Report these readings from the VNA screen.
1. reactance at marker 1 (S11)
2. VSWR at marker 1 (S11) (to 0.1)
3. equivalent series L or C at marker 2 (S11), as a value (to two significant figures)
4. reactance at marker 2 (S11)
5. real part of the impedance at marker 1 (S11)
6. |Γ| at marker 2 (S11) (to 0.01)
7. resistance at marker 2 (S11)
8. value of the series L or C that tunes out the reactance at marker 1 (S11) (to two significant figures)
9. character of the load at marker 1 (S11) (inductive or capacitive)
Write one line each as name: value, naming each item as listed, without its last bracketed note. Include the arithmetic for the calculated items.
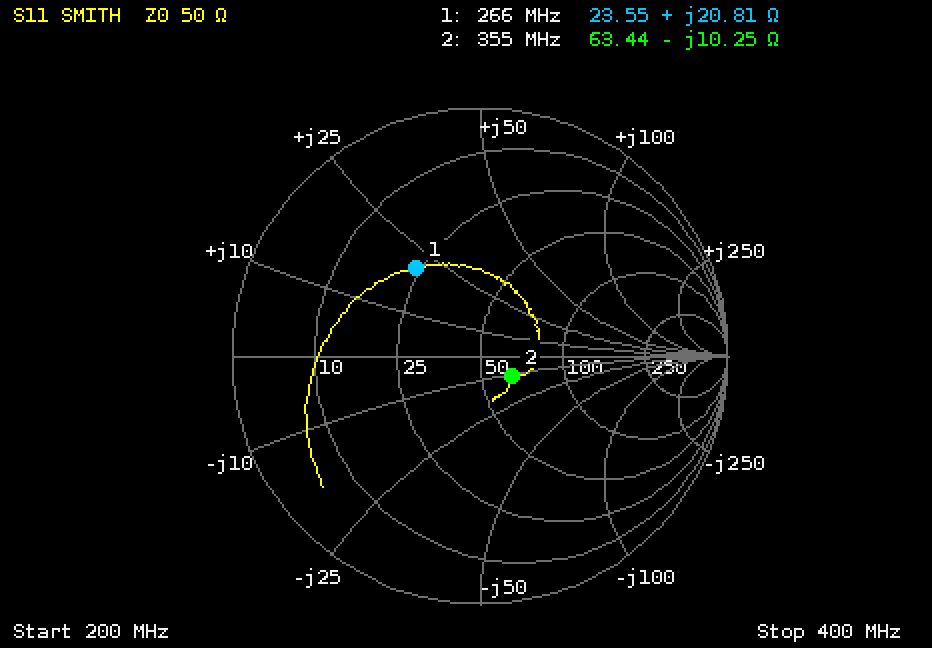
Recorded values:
reactance at marker 1: +20.81 Ω
VSWR at marker 1 (S11): 2.6
equivalent series L or C at marker 2 (S11), as a value: C = 1/(2π × 355 MHz × 10.25 Ω) ≈ 44 pF
reactance at marker 2: -10.25 Ω
real part of the impedance at marker 1: 23.55 Ω
|Γ| at marker 2 (S11): 0.15
resistance at marker 2: 63.44 Ω
value of the series L or C that tunes out the reactance at marker 1 (S11): C = 1/(2π × 266 MHz × 20.81 Ω) ≈ 29 pF
character of the load at marker 1 (S11): inductive
